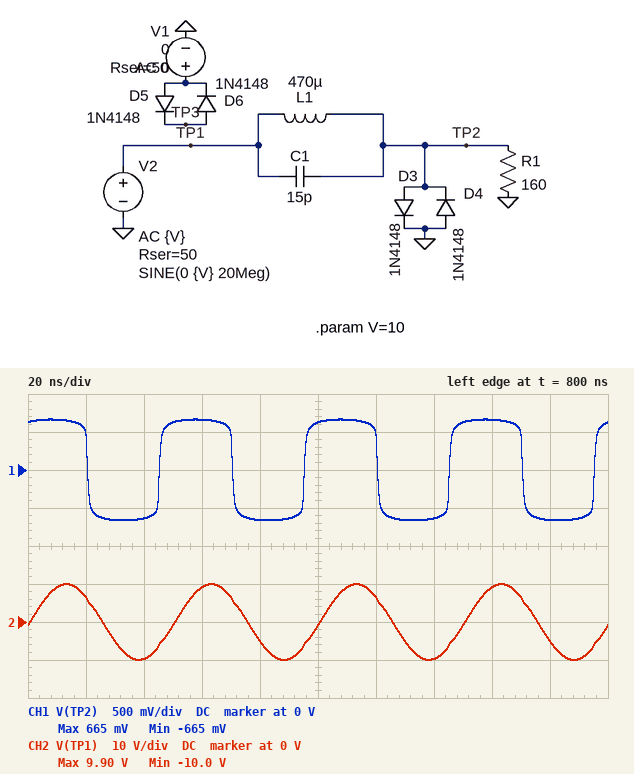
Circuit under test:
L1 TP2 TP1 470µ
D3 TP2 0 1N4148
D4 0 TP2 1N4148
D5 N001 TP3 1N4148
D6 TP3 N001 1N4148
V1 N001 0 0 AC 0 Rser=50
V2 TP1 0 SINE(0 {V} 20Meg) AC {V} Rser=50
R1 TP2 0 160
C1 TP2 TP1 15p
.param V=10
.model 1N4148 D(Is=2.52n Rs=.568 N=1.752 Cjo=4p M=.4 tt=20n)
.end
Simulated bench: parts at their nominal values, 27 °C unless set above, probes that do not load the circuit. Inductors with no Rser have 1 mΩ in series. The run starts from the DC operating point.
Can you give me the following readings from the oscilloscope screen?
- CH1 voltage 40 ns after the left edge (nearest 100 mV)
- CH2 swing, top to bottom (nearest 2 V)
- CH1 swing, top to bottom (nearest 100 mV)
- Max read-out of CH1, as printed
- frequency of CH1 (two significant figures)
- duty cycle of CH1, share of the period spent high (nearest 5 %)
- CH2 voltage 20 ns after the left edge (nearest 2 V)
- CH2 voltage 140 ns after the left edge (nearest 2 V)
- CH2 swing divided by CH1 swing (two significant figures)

-600 mV
20 V
1.3 V
665 mV
20 MHz
50 %
6 V
-10 V
15
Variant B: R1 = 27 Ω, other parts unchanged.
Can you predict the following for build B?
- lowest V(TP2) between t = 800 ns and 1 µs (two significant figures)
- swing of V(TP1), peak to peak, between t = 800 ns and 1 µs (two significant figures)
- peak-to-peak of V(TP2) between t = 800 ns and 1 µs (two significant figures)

-490 mV
20 V
980 mV
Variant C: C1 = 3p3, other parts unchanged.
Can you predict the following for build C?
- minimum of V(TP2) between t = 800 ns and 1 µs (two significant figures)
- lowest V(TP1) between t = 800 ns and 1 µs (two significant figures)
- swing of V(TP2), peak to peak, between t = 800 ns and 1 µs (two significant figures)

-510 mV
-10 V
1.0 V
